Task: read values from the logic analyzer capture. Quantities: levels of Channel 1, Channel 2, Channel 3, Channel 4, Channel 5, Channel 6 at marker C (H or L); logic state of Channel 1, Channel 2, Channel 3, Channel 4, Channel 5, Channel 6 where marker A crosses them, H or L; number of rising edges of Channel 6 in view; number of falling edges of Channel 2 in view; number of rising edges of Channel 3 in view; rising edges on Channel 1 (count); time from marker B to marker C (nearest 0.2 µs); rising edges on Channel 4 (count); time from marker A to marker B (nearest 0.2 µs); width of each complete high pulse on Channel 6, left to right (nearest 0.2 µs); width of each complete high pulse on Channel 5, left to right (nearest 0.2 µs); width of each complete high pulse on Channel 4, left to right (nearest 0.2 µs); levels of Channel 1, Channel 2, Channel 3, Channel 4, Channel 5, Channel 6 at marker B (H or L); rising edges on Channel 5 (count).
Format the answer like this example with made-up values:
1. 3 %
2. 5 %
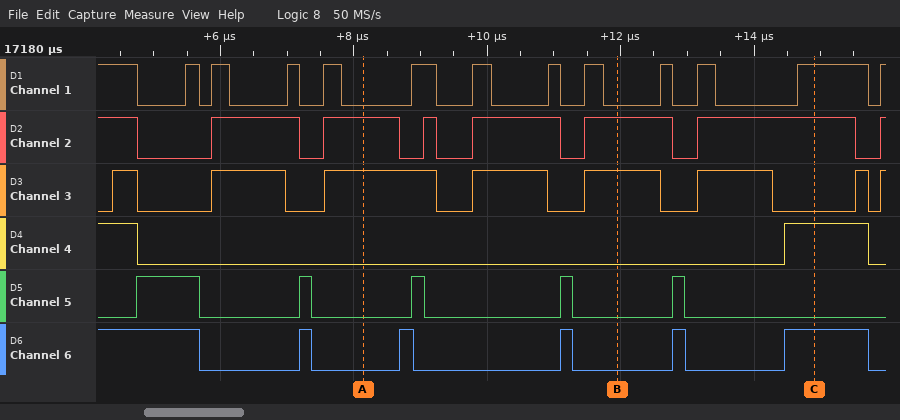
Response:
1. Channel 1=H, Channel 2=H, Channel 3=L, Channel 4=H, Channel 5=L, Channel 6=H
2. Channel 1=L, Channel 2=H, Channel 3=H, Channel 4=L, Channel 5=L, Channel 6=L
3. 5
4. 7
5. 8
6. 12
7. 3 µs
8. 1
9. 3.8 µs
10. 0.2 µs, 0.2 µs, 0.2 µs, 0.2 µs, 1.2 µs
11. 1 µs, 0.2 µs, 0.2 µs, 0.2 µs, 0.2 µs
12. 1.2 µs
13. Channel 1=L, Channel 2=H, Channel 3=H, Channel 4=L, Channel 5=L, Channel 6=L
14. 5
